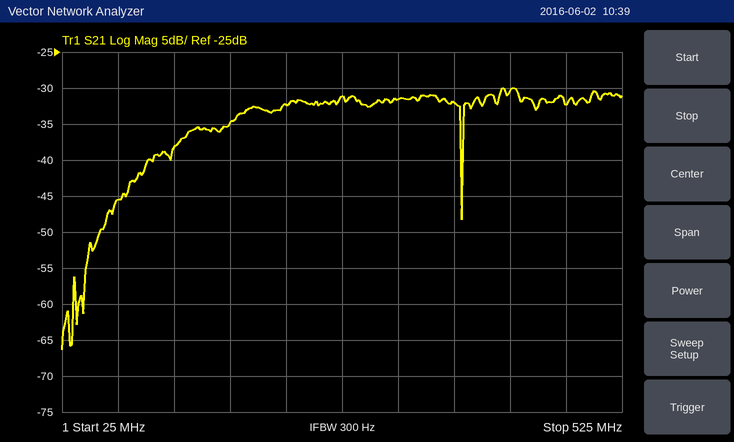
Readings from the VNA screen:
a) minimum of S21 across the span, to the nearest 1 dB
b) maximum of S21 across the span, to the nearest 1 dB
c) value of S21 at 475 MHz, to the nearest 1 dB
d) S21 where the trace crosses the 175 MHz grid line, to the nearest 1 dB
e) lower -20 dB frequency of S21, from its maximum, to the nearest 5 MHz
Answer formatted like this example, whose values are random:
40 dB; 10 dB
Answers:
-66 dB; -30 dB; -32 dB; -35 dB; 60 MHz
